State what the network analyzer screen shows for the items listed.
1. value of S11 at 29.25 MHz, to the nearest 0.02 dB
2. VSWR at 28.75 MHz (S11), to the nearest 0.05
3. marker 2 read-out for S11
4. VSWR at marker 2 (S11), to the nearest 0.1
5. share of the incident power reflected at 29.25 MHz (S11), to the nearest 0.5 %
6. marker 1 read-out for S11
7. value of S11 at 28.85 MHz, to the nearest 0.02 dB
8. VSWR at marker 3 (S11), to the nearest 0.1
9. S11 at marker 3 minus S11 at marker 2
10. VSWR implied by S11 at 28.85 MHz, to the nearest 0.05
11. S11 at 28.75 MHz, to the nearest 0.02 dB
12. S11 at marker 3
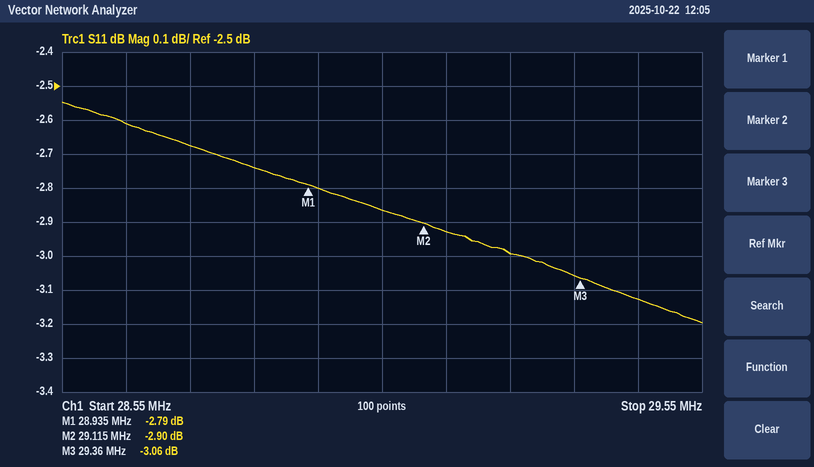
-3.00 dB
6.55
-2.90 dB
6.0
50.0 %
-2.79 dB
-2.74 dB
5.7
-0.16 dB
6.40
-2.68 dB
-3.06 dB
